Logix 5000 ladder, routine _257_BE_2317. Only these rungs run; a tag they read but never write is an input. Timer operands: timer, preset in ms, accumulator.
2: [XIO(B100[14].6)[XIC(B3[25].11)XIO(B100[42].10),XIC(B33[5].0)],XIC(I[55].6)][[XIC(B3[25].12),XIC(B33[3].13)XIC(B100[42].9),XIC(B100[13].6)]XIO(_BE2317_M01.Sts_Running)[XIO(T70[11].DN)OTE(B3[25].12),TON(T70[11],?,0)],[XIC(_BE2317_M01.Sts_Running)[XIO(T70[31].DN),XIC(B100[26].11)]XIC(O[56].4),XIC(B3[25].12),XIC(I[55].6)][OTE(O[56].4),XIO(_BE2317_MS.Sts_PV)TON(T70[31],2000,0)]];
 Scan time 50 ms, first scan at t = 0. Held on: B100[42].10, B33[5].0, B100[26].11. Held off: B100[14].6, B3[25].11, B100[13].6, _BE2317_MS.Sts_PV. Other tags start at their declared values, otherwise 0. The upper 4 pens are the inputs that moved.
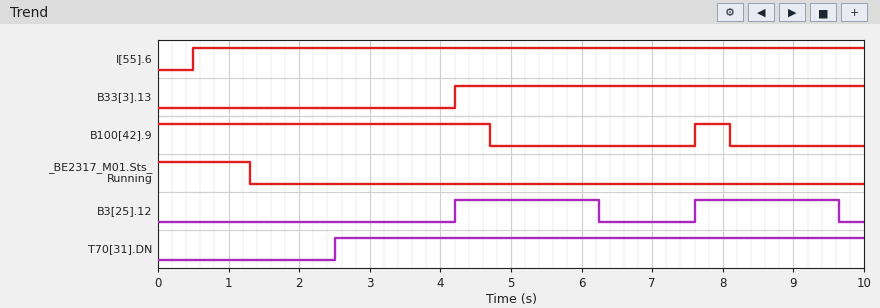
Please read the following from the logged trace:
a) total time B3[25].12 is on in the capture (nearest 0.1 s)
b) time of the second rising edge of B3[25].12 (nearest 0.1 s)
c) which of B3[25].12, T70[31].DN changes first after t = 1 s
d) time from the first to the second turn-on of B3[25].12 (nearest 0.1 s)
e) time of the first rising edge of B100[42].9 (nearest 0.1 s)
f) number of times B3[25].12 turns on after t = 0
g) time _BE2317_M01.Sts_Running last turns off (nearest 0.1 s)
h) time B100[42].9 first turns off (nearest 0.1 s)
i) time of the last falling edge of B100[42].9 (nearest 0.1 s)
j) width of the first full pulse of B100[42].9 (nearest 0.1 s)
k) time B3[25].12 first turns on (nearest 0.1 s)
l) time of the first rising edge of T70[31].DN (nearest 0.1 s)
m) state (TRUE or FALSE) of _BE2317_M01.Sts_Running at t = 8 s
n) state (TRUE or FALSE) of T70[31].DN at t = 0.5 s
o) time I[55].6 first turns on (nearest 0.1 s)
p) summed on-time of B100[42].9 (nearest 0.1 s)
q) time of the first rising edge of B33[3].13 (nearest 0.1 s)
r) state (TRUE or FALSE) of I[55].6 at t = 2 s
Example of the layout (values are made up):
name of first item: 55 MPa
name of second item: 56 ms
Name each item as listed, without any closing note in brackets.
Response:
total time B3[25].12 is on in the capture: 4.1 s
time of the second rising edge of B3[25].12: 7.6 s
which of B3[25].12, T70[31].DN changes first after t = 1 s: T70[31].DN
time from the first to the second turn-on of B3[25].12: 3.4 s
time of the first rising edge of B100[42].9: 7.6 s
number of times B3[25].12 turns on after t = 0: 2
time _BE2317_M01.Sts_Running last turns off: 1.3 s
time B100[42].9 first turns off: 4.7 s
time of the last falling edge of B100[42].9: 8.1 s
width of the first full pulse of B100[42].9: 0.5 s
time B3[25].12 first turns on: 4.2 s
time of the first rising edge of T70[31].DN: 2.5 s
state (TRUE or FALSE) of _BE2317_M01.Sts_Running at t = 8 s: FALSE
state (TRUE or FALSE) of T70[31].DN at t = 0.5 s: FALSE
time I[55].6 first turns on: 0.5 s
summed on-time of B100[42].9: 5.2 s
time of the first rising edge of B33[3].13: 4.2 s
state (TRUE or FALSE) of I[55].6 at t = 2 s: TRUE
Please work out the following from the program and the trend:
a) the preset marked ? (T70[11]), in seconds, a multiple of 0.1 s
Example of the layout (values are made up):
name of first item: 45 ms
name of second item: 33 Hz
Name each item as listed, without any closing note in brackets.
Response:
the preset marked ? (T70[11]), in seconds, a multiple of 0.1 s: 2.0 s
